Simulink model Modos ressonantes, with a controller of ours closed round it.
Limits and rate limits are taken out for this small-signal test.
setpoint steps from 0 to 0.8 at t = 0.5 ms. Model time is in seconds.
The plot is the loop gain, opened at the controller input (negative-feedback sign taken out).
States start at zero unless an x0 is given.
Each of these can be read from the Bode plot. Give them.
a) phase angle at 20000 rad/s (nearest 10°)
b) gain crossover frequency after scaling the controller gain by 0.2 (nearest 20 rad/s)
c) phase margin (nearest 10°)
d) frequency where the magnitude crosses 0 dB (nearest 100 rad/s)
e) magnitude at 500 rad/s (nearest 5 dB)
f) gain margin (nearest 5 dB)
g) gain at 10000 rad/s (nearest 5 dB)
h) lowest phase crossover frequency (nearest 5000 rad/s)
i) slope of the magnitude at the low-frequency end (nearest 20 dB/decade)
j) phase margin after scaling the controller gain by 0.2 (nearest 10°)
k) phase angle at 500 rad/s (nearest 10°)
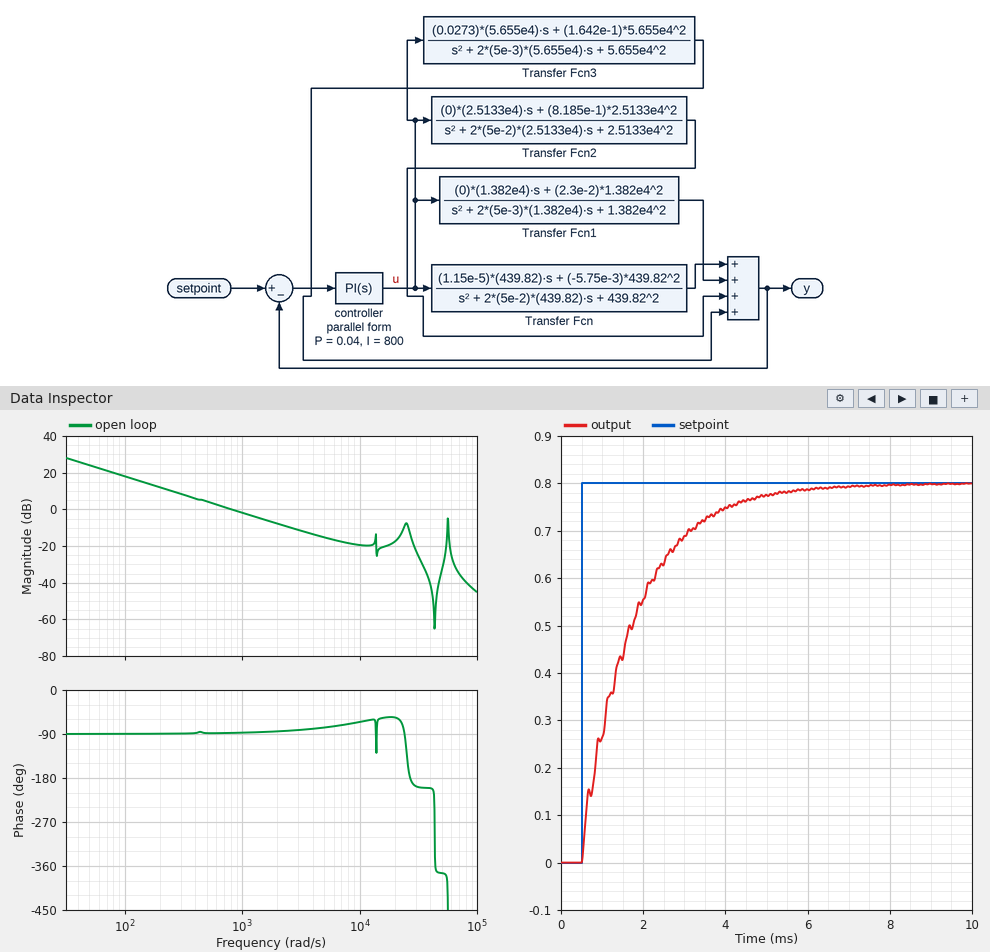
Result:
-60°
160 rad/s
90°
800 rad/s
5 dB
15 dB
-20 dB
25000 rad/s
-20 dB/decade
90°
-90°
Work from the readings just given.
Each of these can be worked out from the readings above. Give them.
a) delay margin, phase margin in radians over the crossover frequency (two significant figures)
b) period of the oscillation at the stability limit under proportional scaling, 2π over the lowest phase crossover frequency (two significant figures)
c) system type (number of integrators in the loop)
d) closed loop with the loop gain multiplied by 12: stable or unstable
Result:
0.0020 s
0.00025 s
1
unstable
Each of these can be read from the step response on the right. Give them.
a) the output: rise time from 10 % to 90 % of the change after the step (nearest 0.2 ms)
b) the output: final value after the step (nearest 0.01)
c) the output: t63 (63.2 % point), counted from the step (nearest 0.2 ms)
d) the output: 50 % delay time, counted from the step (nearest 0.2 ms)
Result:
2.8 ms
0.80
1.2 ms
0.8 ms
